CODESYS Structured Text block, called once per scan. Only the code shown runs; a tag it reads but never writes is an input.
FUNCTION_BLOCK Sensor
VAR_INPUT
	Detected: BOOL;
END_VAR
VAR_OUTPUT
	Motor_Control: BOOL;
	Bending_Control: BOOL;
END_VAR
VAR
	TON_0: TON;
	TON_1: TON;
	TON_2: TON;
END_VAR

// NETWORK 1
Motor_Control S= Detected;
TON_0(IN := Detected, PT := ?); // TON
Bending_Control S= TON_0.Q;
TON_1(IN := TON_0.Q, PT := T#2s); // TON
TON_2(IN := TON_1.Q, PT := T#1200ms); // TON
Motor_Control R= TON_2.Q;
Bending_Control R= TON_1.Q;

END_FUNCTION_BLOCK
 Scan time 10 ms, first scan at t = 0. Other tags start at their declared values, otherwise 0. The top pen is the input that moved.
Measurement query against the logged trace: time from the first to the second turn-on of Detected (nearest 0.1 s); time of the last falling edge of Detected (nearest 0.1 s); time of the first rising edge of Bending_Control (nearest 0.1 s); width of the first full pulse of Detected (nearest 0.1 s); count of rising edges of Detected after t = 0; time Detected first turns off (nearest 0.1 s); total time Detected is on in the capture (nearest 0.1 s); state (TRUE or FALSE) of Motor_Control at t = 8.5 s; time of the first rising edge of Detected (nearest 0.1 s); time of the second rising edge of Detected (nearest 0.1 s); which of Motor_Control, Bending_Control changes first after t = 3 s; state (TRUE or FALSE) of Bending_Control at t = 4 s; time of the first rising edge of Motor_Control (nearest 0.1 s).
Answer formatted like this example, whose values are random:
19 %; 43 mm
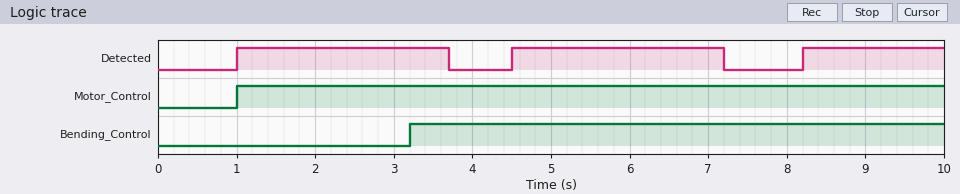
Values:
3.5 s; 7.2 s; 3.2 s; 2.7 s; 3; 3.7 s; 7.2 s; TRUE; 1.0 s; 4.5 s; Bending_Control; TRUE; 1.0 s
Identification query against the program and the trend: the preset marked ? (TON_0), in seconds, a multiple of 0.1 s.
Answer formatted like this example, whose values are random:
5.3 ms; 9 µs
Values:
2.2 s
